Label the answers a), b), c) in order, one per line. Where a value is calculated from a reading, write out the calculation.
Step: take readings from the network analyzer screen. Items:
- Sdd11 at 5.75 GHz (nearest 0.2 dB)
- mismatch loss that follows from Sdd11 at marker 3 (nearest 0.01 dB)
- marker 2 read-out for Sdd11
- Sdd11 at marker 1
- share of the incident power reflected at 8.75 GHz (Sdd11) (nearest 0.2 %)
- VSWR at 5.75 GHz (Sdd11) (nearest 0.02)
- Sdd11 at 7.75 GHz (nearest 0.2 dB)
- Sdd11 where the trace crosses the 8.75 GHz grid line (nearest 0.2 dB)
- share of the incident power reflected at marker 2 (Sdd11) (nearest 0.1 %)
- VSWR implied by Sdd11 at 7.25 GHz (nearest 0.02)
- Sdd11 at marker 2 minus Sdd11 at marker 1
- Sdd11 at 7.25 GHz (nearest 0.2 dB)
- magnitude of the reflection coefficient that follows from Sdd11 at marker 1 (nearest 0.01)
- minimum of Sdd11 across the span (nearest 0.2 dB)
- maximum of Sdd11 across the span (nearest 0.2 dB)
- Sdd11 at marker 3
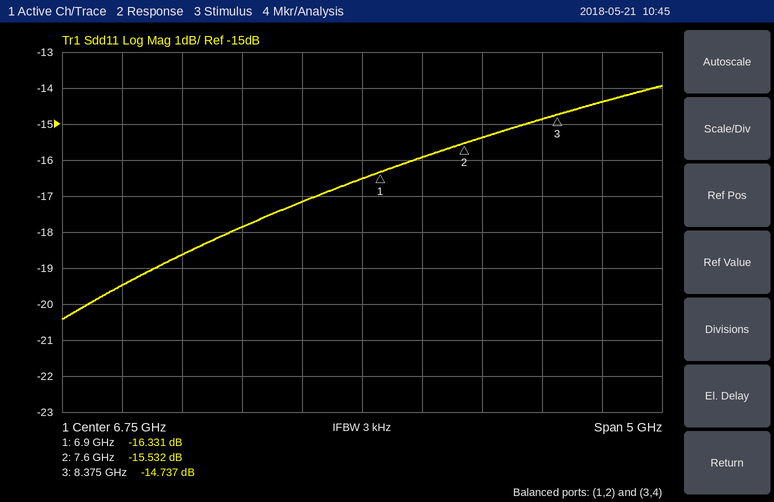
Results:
a) -17.8 dB
b) −10 log10(1 − 10^(-14.737/10)) ≈ 0.15 dB
c) -15.532 dB
d) -16.331 dB
e) 10^(-14.4/10) ≈ 3.6 %
f) |Γ| = 10^(-17.8/20) = 0.1288; VSWR = (1 + 0.1288)/(1 − 0.1288) ≈ 1.30
g) -15.4 dB
h) -14.4 dB
i) 10^(-15.532/10) ≈ 2.8 %
j) |Γ| = 10^(-16/20) = 0.1585; VSWR = (1 + 0.1585)/(1 − 0.1585) ≈ 1.38
k) -15.532 − (-16.331) = 0.799 dB
l) -16.0 dB
m) 10^(-16.331/20) ≈ 0.15
n) -20.4 dB
o) -14.0 dB
p) -14.737 dB
